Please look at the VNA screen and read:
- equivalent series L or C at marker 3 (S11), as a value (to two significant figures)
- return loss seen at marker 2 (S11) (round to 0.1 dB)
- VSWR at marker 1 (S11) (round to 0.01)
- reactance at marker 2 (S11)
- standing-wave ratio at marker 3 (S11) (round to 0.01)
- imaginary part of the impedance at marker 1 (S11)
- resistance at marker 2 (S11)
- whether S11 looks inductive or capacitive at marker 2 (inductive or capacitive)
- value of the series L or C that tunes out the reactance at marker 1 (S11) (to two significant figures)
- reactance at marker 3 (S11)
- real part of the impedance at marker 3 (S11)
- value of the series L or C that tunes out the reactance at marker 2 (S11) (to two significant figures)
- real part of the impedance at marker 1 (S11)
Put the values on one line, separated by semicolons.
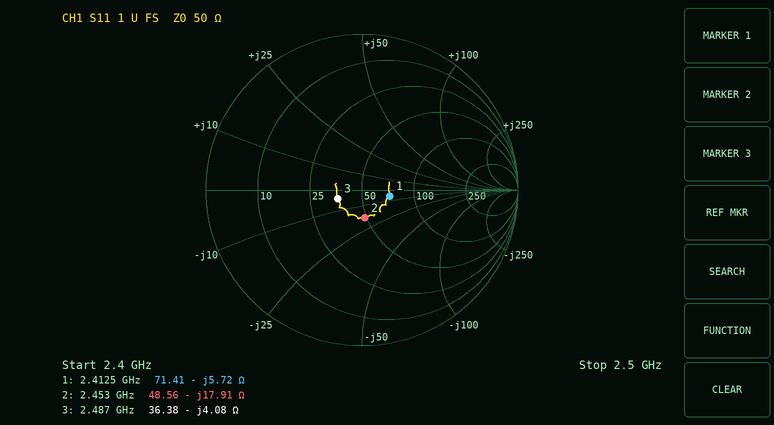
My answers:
16 pF; 14.9 dB; 1.45; -17.91 Ω; 1.39; -5.72 Ω; 48.56 Ω; capacitive; 380 pH; -4.08 Ω; 36.38 Ω; 1.2 nH; 71.41 Ω
